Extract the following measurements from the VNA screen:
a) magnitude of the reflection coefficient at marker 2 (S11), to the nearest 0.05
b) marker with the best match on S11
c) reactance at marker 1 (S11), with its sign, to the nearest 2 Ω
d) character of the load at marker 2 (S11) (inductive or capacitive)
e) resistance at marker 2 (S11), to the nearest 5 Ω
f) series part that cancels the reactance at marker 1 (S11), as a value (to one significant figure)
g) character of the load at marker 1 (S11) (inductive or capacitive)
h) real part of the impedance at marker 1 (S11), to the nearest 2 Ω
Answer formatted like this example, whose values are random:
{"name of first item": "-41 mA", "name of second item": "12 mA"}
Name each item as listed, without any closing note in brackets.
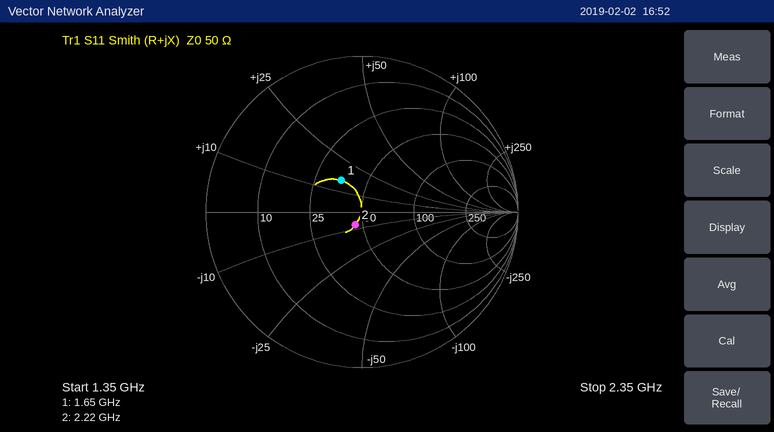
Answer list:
{"magnitude of the reflection coefficient at marker 2 (S11), to the nearest 0.05": "0.10", "marker with the best match on S11": "marker 2", "reactance at marker 1 (S11), with its sign, to the nearest 2 Ω": "+16 Ω", "character of the load at marker 2 (S11)": "capacitive", "resistance at marker 2 (S11), to the nearest 5 Ω": "45 Ω", "series part that cancels the reactance at marker 1 (S11), as a value": "6 pF", "character of the load at marker 1 (S11)": "inductive", "real part of the impedance at marker 1 (S11), to the nearest 2 Ω": "36 Ω"}
